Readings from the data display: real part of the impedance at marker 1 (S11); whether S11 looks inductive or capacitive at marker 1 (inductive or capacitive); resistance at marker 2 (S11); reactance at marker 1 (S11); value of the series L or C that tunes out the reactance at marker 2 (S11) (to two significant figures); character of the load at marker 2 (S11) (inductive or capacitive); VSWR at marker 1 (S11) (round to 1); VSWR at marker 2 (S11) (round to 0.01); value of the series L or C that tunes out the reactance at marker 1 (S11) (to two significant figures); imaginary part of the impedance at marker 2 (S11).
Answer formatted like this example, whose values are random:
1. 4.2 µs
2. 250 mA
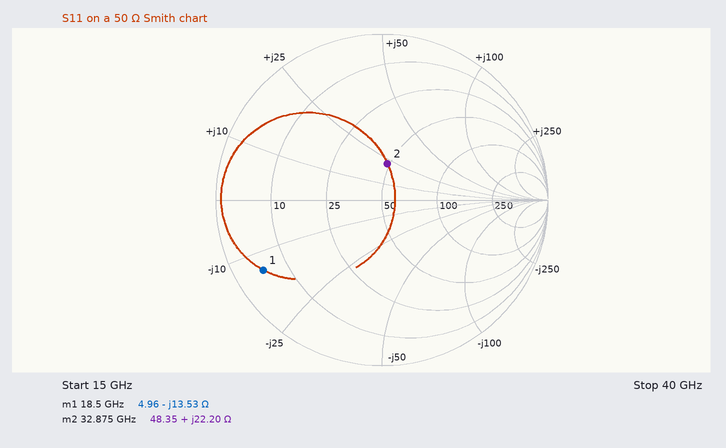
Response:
1. 4.96 Ω
2. capacitive
3. 48.35 Ω
4. -13.53 Ω
5. 220 fF
6. inductive
7. 11
8. 1.57
9. 120 pH
10. +22.20 Ω
